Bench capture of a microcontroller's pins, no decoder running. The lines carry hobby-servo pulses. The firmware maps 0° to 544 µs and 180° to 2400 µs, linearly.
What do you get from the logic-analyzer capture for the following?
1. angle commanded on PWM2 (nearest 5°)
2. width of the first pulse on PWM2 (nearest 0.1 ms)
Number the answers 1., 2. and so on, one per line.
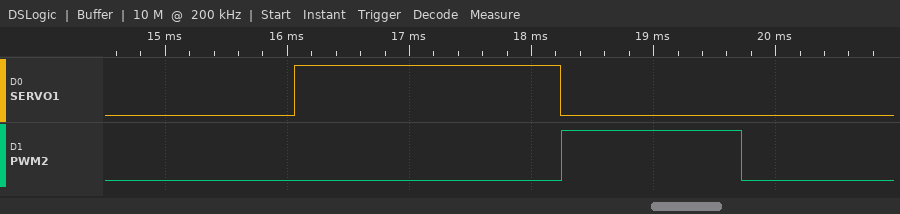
1. 90°
2. 1.5 ms
